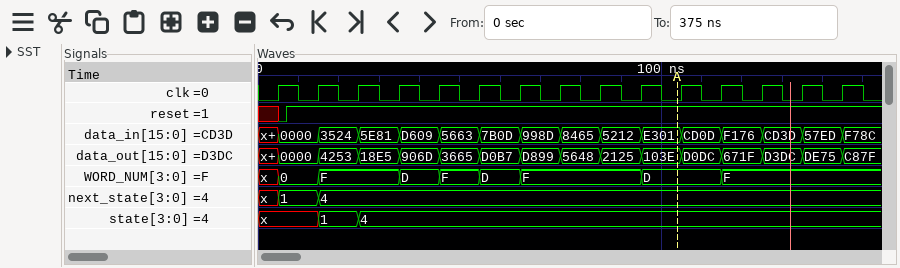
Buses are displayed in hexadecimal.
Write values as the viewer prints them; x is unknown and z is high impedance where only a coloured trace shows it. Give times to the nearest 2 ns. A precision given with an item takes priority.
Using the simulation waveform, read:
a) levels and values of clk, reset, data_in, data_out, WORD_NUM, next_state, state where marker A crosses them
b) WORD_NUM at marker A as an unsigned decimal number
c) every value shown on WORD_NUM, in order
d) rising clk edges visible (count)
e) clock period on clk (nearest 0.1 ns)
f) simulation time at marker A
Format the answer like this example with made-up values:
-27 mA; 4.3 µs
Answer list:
clk=0, reset=1, data_in=E301, data_out=103E, WORD_NUM=D, next_state=4, state=4; 13; x, 0, F, D, F, D, F, D, F; 15; 10 ns; 104 ns
